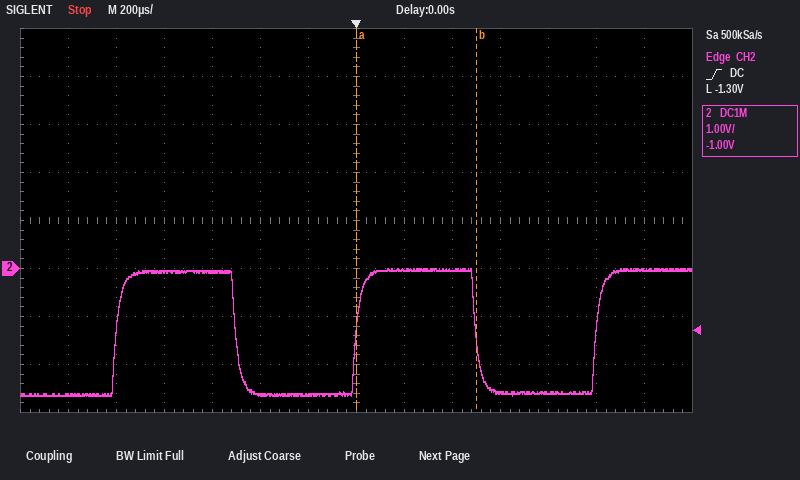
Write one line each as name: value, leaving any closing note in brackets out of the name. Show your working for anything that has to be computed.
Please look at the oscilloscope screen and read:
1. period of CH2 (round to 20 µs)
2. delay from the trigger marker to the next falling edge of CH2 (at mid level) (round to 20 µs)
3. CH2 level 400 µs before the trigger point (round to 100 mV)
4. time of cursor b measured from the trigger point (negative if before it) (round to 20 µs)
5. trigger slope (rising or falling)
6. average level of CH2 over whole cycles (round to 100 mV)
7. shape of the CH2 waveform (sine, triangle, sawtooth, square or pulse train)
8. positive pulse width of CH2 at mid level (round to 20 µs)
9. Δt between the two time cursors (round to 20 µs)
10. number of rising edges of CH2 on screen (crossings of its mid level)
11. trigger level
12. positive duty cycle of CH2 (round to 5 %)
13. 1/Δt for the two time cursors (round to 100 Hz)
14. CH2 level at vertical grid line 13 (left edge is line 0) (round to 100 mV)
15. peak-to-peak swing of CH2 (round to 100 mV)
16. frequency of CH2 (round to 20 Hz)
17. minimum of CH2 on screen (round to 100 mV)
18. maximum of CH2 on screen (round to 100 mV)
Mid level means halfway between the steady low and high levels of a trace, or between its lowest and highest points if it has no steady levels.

period of CH2: 1.00 ms
delay from the trigger marker to the next falling edge of CH2 (at mid level): 500 µs
CH2 level 400 µs before the trigger point: -2.6 V
time of cursor b measured from the trigger point (negative if before it): +500 µs
trigger slope: rising
average level of CH2 over whole cycles: -2.6 V + 0.5 × (0.0 V − (-2.6 V)) ≈ -1.3 V
shape of the CH2 waveform: square
positive pulse width of CH2 at mid level: 500 µs
Δt between the two time cursors: 500 µs
number of rising edges of CH2 on screen: 3
trigger level: -1.30 V
positive duty cycle of CH2: 500 µs / 1.00 ms ≈ 50 %
1/Δt for the two time cursors: 1 / 500 µs ≈ 2.0 kHz
CH2 level at vertical grid line 13 (left edge is line 0): 0.0 V
peak-to-peak swing of CH2: 0.0 V − (-2.6 V) = 2.6 V
frequency of CH2: 1 / 1.00 ms ≈ 1.00 kHz
minimum of CH2 on screen: -2.6 V
maximum of CH2 on screen: 0.0 V
